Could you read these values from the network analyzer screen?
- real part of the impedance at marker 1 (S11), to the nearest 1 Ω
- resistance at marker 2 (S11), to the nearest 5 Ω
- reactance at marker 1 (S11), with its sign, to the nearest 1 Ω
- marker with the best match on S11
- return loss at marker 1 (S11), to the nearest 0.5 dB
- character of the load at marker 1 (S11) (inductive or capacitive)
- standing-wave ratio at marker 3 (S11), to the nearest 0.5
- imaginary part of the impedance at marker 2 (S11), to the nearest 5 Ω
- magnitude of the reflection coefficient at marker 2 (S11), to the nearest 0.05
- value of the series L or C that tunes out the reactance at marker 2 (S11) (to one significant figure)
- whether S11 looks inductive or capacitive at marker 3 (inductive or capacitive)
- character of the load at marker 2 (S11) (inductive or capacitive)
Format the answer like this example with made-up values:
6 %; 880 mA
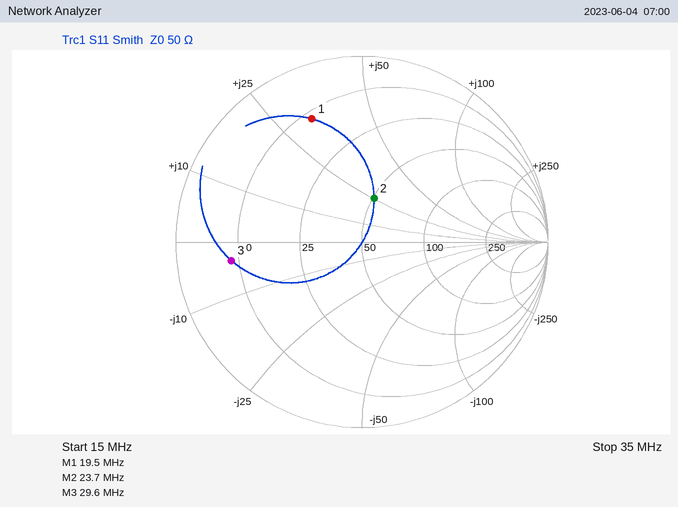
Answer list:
12 Ω; 50 Ω; +32 Ω; marker 2; 3.0 dB; inductive; 6.0; +25 Ω; 0.25; 300 pF; capacitive; inductive
